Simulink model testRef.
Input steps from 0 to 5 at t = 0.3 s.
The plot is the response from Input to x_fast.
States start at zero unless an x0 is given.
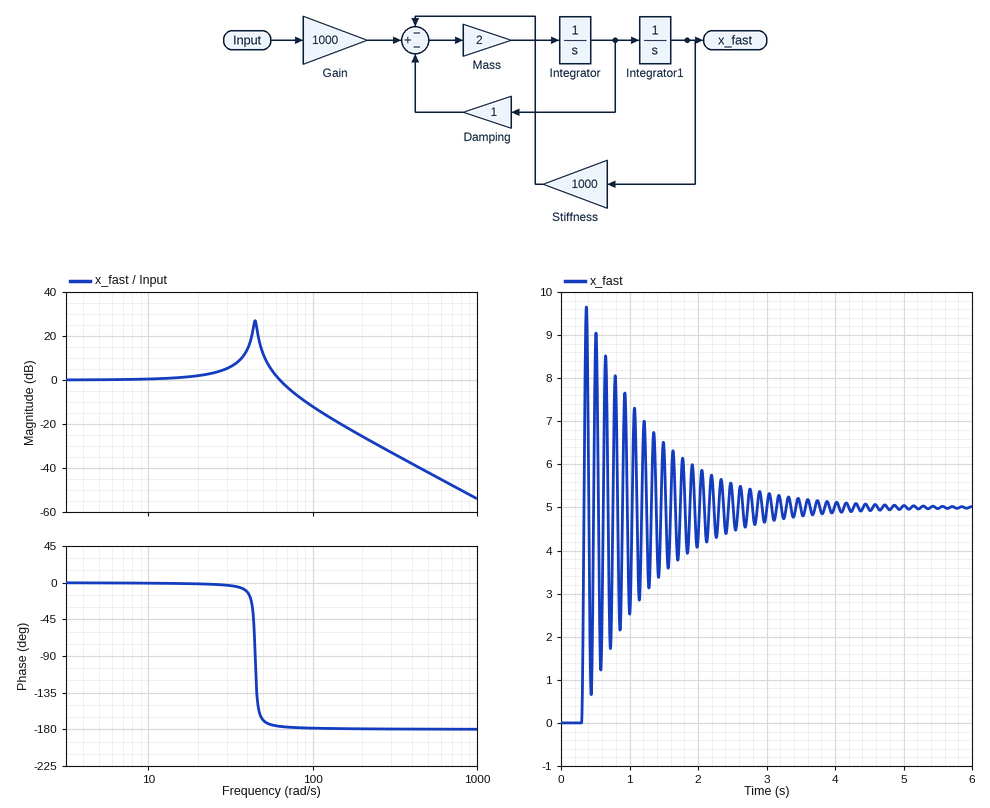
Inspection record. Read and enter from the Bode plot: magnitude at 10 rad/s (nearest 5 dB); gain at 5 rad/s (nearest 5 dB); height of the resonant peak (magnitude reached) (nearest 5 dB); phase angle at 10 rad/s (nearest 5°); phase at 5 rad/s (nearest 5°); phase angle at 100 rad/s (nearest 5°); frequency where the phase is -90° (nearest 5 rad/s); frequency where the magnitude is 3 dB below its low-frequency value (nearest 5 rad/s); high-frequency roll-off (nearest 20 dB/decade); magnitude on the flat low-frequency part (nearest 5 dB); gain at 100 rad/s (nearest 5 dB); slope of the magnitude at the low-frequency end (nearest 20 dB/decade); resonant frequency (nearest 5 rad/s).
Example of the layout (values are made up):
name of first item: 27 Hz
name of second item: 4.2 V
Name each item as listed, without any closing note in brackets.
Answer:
magnitude at 10 rad/s: 0 dB
gain at 5 rad/s: 0 dB
height of the resonant peak (magnitude reached): 25 dB
phase angle at 10 rad/s: 0°
phase at 5 rad/s: 0°
phase angle at 100 rad/s: -180°
frequency where the phase is -90°: 45 rad/s
frequency where the magnitude is 3 dB below its low-frequency value: 70 rad/s
high-frequency roll-off: -40 dB/decade
magnitude on the flat low-frequency part: 0 dB
gain at 100 rad/s: -10 dB
slope of the magnitude at the low-frequency end: 0 dB/decade
resonant frequency: 45 rad/s
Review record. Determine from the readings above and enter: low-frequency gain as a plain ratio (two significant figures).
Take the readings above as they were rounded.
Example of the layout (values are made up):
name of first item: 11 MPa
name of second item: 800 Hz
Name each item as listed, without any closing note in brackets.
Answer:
low-frequency gain as a plain ratio: 1.0
